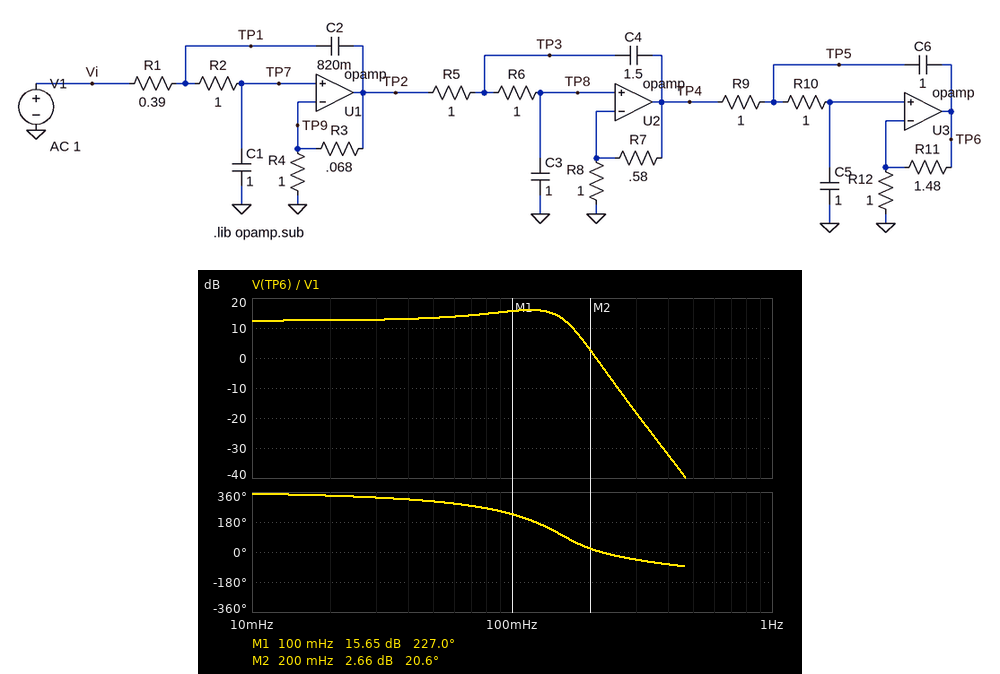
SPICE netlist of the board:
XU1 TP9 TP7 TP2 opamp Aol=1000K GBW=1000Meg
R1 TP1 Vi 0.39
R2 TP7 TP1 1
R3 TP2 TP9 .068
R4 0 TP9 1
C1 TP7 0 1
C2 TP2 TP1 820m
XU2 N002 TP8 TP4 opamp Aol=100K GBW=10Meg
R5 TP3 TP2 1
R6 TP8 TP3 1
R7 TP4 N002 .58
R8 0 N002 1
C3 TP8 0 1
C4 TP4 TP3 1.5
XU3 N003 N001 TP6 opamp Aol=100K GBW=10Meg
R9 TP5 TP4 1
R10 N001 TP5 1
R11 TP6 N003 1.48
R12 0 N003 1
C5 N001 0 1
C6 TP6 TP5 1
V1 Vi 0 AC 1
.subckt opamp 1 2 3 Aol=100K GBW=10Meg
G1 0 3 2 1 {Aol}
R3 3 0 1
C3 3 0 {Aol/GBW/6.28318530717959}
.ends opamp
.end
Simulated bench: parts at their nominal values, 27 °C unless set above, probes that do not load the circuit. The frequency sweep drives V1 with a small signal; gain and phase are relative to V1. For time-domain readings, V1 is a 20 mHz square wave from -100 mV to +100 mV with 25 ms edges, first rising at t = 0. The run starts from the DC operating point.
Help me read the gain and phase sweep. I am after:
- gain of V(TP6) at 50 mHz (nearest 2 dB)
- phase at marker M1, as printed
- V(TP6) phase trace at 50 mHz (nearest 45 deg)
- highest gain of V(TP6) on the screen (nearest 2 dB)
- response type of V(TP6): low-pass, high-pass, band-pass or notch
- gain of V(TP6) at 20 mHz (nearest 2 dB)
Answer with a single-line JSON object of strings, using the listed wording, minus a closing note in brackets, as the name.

{"gain of V(TP6) at 50 mHz": "14 dB", "phase at marker M1, as printed": "227.0 deg", "V(TP6) phase trace at 50 mHz": "315 deg", "highest gain of V(TP6) on the screen": "16 dB", "response type of V(TP6): low-pass, high-pass, band-pass or notch": "low-pass", "gain of V(TP6) at 20 mHz": "12 dB"}
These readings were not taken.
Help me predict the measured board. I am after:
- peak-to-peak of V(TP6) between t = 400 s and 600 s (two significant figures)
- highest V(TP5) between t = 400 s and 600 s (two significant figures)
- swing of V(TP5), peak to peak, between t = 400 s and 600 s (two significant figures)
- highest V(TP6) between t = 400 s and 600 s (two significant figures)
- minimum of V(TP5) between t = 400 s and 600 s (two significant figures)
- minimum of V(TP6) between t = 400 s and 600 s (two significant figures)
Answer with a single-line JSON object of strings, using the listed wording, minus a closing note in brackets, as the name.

{"peak-to-peak of V(TP6) between t = 400 s and 600 s": "1.4 V", "highest V(TP5) between t = 400 s and 600 s": "330 mV", "swing of V(TP5), peak to peak, between t = 400 s and 600 s": "660 mV", "highest V(TP6) between t = 400 s and 600 s": "710 mV", "minimum of V(TP5) between t = 400 s and 600 s": "-330 mV", "minimum of V(TP6) between t = 400 s and 600 s": "-710 mV"}
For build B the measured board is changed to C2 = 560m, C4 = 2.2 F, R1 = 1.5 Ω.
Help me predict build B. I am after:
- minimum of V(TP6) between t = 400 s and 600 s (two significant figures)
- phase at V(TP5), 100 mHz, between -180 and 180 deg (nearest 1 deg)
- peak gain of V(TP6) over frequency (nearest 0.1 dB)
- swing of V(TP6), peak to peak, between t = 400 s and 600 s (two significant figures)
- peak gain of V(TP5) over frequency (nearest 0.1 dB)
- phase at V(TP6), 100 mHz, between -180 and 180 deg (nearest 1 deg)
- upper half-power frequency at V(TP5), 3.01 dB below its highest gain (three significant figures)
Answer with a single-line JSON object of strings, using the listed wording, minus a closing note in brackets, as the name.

{"minimum of V(TP6) between t = 400 s and 600 s": "-740 mV", "phase at V(TP5), 100 mHz, between -180 and 180 deg": "-137 deg", "peak gain of V(TP6) over frequency": "17.7 dB", "swing of V(TP6), peak to peak, between t = 400 s and 600 s": "1.5 V", "peak gain of V(TP5) over frequency": "11.3 dB", "phase at V(TP6), 100 mHz, between -180 and 180 deg": "-169 deg", "upper half-power frequency at V(TP5), 3.01 dB below its highest gain": "130 mHz"}
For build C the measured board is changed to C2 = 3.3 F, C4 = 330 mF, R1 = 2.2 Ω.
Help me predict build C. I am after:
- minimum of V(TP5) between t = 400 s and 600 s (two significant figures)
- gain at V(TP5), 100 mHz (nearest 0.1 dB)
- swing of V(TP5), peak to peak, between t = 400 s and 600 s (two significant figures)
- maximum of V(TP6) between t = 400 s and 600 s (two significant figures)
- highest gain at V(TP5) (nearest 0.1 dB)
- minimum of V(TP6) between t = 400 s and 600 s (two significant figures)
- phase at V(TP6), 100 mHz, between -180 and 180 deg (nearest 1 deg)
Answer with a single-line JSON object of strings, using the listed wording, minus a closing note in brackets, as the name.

{"minimum of V(TP5) between t = 400 s and 600 s": "-220 mV", "gain at V(TP5), 100 mHz": "-1.9 dB", "swing of V(TP5), peak to peak, between t = 400 s and 600 s": "440 mV", "maximum of V(TP6) between t = 400 s and 600 s": "540 mV", "highest gain at V(TP5)": "5.9 dB", "minimum of V(TP6) between t = 400 s and 600 s": "-540 mV", "phase at V(TP6), 100 mHz, between -180 and 180 deg": "141 deg"}
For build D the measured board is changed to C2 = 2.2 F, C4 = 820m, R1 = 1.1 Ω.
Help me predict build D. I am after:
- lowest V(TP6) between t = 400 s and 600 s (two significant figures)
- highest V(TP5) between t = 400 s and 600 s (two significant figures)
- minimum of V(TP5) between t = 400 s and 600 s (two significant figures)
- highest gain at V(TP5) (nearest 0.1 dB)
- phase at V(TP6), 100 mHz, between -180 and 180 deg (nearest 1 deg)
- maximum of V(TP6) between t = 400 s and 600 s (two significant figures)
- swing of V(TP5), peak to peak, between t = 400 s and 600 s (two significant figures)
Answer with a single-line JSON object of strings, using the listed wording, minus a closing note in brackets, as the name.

{"lowest V(TP6) between t = 400 s and 600 s": "-580 mV", "highest V(TP5) between t = 400 s and 600 s": "260 mV", "minimum of V(TP5) between t = 400 s and 600 s": "-260 mV", "highest gain at V(TP5)": "6.3 dB", "phase at V(TP6), 100 mHz, between -180 and 180 deg": "-171 deg", "maximum of V(TP6) between t = 400 s and 600 s": "580 mV", "swing of V(TP5), peak to peak, between t = 400 s and 600 s": "520 mV"}
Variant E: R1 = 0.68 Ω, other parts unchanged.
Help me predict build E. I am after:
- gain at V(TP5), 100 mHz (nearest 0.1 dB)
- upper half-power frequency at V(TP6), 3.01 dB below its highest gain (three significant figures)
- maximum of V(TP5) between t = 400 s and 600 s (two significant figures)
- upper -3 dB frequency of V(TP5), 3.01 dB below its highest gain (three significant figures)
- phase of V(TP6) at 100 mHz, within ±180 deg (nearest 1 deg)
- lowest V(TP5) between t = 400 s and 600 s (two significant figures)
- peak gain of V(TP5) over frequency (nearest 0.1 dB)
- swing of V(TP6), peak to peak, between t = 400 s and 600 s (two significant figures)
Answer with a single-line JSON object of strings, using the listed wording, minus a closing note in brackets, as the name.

{"gain at V(TP5), 100 mHz": "8.7 dB", "upper half-power frequency at V(TP6), 3.01 dB below its highest gain": "155 mHz", "maximum of V(TP5) between t = 400 s and 600 s": "320 mV", "upper -3 dB frequency of V(TP5), 3.01 dB below its highest gain": "161 mHz", "phase of V(TP6) at 100 mHz, within ±180 deg": "-141 deg", "lowest V(TP5) between t = 400 s and 600 s": "-320 mV", "peak gain of V(TP5) over frequency": "9.5 dB", "swing of V(TP6), peak to peak, between t = 400 s and 600 s": "1.4 V"}
